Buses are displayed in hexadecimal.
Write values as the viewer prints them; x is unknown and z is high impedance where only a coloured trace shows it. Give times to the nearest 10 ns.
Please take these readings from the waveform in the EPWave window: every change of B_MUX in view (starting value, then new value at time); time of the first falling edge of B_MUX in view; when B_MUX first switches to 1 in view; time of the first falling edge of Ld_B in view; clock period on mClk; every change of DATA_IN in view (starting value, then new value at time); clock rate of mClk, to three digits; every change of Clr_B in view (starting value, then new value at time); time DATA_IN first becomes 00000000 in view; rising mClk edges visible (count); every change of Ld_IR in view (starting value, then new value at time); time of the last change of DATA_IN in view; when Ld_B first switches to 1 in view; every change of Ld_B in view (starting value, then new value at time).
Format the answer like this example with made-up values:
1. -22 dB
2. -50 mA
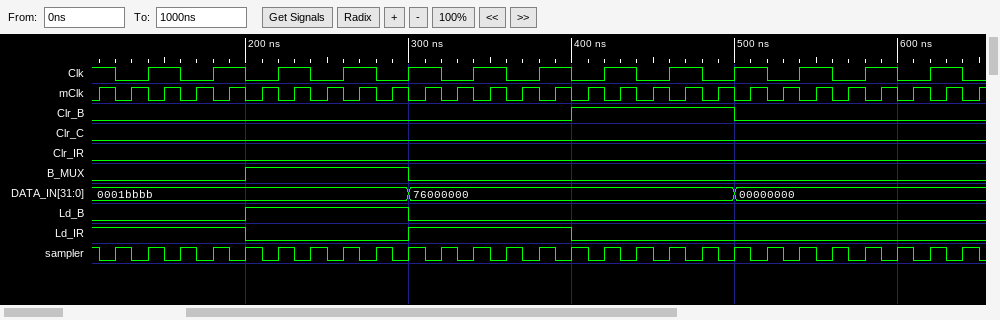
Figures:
1. 0, 1 at 200 ns, 0 at 300 ns
2. 300 ns
3. 200 ns
4. 300 ns
5. 20 ns
6. 0001bbbb, 76000000 at 300 ns, 00000000 at 500 ns
7. 50.0 MHz
8. 0, 1 at 400 ns, 0 at 500 ns
9. 500 ns
10. 28
11. 1, 0 at 200 ns, 1 at 300 ns, 0 at 400 ns
12. 500 ns
13. 200 ns
14. 0, 1 at 200 ns, 0 at 300 ns
